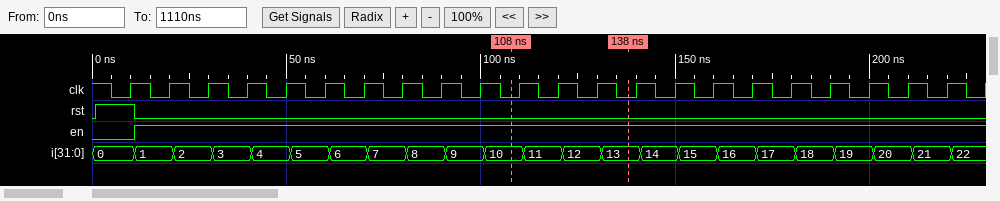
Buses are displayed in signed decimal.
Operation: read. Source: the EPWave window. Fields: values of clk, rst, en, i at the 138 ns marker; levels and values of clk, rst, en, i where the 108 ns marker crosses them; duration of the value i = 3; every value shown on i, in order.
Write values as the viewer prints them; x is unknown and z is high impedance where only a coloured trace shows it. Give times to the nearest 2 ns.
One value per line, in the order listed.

clk=0, rst=0, en=1, i=13
clk=0, rst=0, en=1, i=10
10 ns
0, 1, 2, 3, 4, 5, 6, 7, 8, 9, 10, 11, 12, 13, 14, 15, 16, 17, 18, 19, 20, 21, 22
